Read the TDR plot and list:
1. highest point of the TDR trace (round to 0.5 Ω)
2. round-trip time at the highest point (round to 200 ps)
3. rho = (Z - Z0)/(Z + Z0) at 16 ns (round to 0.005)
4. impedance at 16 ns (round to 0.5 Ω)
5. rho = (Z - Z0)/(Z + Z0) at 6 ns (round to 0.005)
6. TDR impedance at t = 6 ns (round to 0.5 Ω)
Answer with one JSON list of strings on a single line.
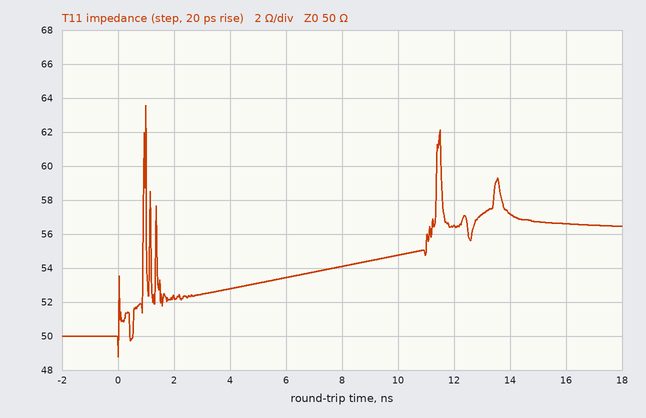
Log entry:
["63.5 Ω", "1.0 ns", "+0.060", "56.5 Ω", "+0.035", "53.5 Ω"]
